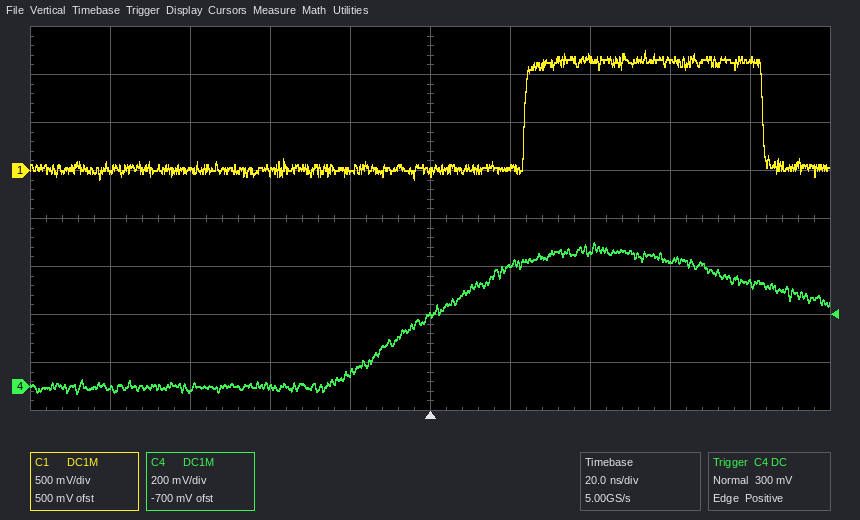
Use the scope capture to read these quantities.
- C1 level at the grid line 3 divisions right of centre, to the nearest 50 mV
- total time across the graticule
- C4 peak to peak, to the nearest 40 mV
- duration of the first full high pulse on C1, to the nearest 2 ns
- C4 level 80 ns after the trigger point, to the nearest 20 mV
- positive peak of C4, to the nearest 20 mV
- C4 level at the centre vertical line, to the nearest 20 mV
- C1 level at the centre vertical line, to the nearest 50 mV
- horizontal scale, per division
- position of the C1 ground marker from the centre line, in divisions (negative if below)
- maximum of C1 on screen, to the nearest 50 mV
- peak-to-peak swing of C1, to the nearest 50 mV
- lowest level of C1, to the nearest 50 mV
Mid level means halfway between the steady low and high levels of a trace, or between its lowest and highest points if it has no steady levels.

1.15 V
200 ns
640 mV
60 ns
420 mV
600 mV
300 mV
0 mV
20 ns
+1.0 div
1.25 V
1.35 V
-100 mV
